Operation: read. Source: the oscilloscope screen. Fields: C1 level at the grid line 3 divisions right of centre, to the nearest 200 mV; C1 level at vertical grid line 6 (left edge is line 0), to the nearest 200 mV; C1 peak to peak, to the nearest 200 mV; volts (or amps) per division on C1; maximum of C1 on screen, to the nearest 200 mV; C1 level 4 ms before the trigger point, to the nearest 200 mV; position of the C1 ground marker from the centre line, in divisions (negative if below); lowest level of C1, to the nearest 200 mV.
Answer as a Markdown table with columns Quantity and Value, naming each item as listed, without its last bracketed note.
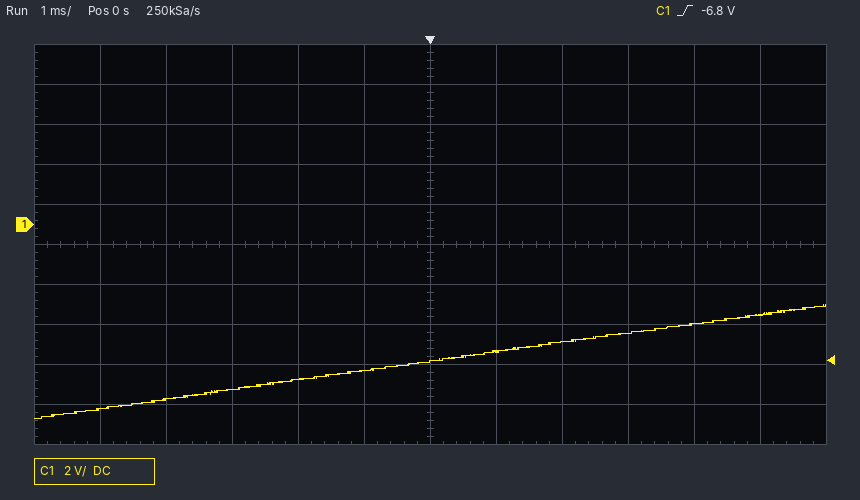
| Quantity | Value |
|---|---|
| C1 level at the grid line 3 divisions right of centre, to the nearest 200 mV | -5.4 V |
| C1 level at vertical grid line 6 (left edge is line 0), to the nearest 200 mV | -6.8 V |
| C1 peak to peak, to the nearest 200 mV | 5.6 V |
| volts (or amps) per division on C1 | 2 V |
| maximum of C1 on screen, to the nearest 200 mV | -4.0 V |
| C1 level 4 ms before the trigger point, to the nearest 200 mV | -8.8 V |
| position of the C1 ground marker from the centre line, in divisions | +0.5 div |
| lowest level of C1, to the nearest 200 mV | -9.6 V |
